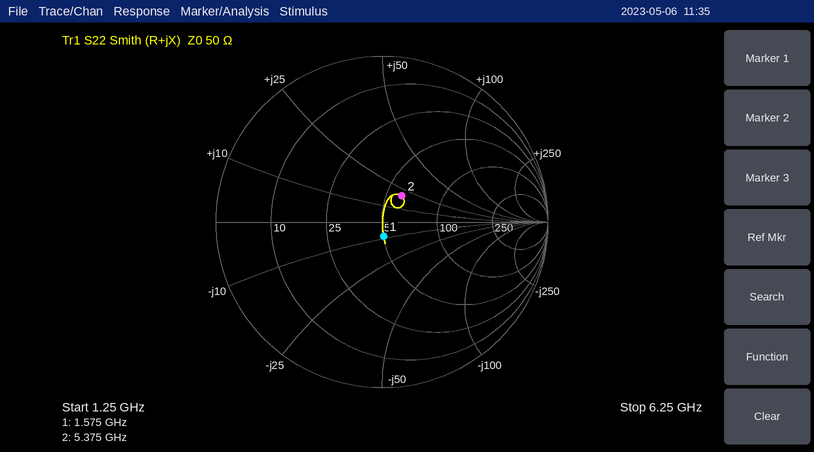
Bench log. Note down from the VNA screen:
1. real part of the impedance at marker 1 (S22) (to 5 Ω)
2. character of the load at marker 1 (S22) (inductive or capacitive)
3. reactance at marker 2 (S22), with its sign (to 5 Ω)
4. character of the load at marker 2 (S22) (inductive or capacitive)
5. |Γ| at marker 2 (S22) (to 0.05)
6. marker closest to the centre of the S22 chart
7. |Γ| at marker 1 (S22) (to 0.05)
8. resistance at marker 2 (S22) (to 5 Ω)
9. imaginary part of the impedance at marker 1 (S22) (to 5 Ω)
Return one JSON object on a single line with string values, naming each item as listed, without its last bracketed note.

{"real part of the impedance at marker 1 (S22)": "50 Ω", "character of the load at marker 1 (S22)": "capacitive", "reactance at marker 2 (S22), with its sign": "+20 Ω", "character of the load at marker 2 (S22)": "inductive", "|Γ| at marker 2 (S22)": "0.20", "marker closest to the centre of the S22 chart": "marker 1", "|Γ| at marker 1 (S22)": "0.10", "resistance at marker 2 (S22)": "60 Ω", "imaginary part of the impedance at marker 1 (S22)": "-10 Ω"}
